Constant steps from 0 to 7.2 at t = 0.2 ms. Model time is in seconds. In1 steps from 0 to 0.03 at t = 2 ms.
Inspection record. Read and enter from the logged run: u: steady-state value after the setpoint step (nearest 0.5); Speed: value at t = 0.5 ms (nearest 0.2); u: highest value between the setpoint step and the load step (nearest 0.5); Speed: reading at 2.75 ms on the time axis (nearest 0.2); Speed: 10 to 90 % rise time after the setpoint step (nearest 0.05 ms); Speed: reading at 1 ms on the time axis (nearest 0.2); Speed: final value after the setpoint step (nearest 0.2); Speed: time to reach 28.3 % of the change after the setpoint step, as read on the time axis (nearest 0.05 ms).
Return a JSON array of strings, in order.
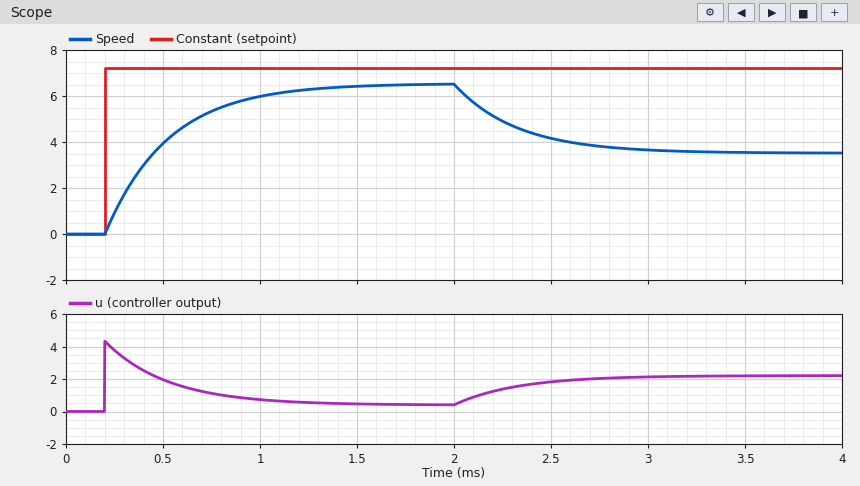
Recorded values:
["0.5", "4.0", "4.5", "3.8", "0.70 ms", "6.0", "6.6", "0.30 ms"]
